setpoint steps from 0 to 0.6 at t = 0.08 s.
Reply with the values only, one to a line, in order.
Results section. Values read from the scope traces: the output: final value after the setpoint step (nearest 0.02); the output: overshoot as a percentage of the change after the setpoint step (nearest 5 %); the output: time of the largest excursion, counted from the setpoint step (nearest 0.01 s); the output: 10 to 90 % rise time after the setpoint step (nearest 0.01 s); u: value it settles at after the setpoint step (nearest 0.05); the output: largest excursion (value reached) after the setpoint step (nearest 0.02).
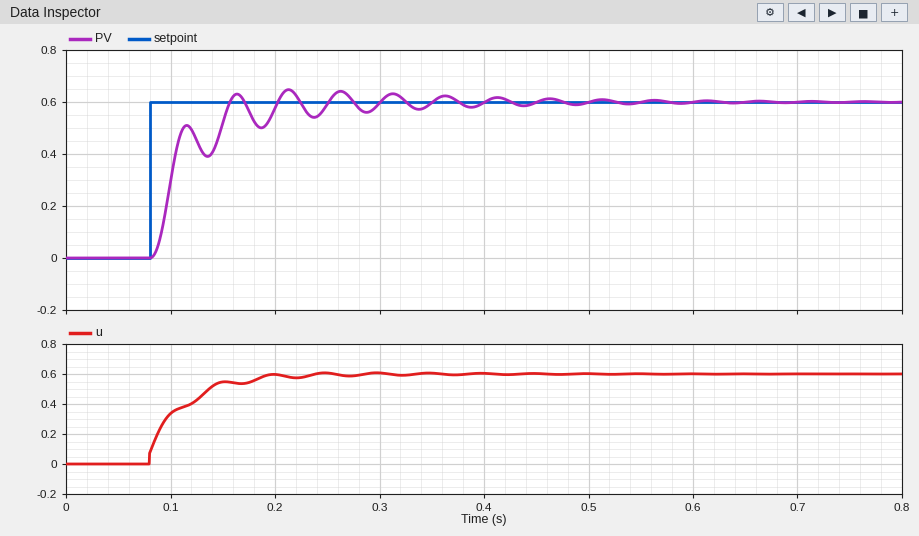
0.60
10 %
0.13 s
0.06 s
0.60
0.64
